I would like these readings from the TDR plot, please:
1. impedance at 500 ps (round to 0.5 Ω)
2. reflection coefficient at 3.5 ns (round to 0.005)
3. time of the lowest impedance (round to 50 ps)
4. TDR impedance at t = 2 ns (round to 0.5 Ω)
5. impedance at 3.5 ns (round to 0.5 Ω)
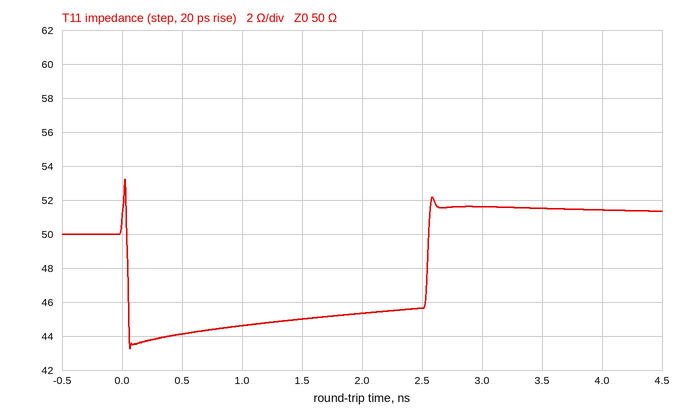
44.0 Ω
+0.015
50 ps
45.5 Ω
51.5 Ω
